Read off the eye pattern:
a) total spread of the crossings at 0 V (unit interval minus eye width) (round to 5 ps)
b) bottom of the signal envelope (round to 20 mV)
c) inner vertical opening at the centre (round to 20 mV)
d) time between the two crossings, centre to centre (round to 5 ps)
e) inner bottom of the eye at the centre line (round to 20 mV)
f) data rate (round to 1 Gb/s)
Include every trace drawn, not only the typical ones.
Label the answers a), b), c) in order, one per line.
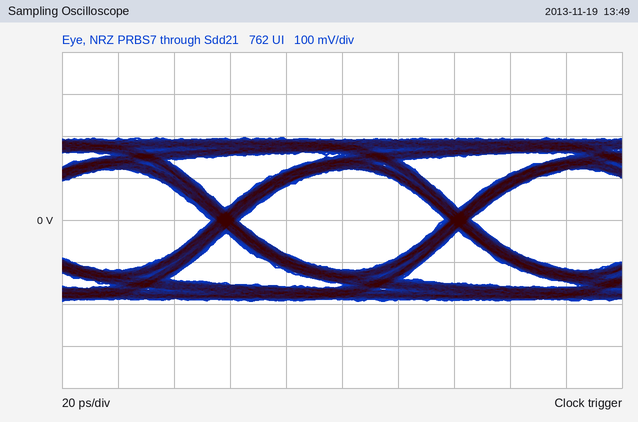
a) 10 ps
b) -200 mV
c) 240 mV
d) 85 ps
e) -120 mV
f) 12 Gb/s
